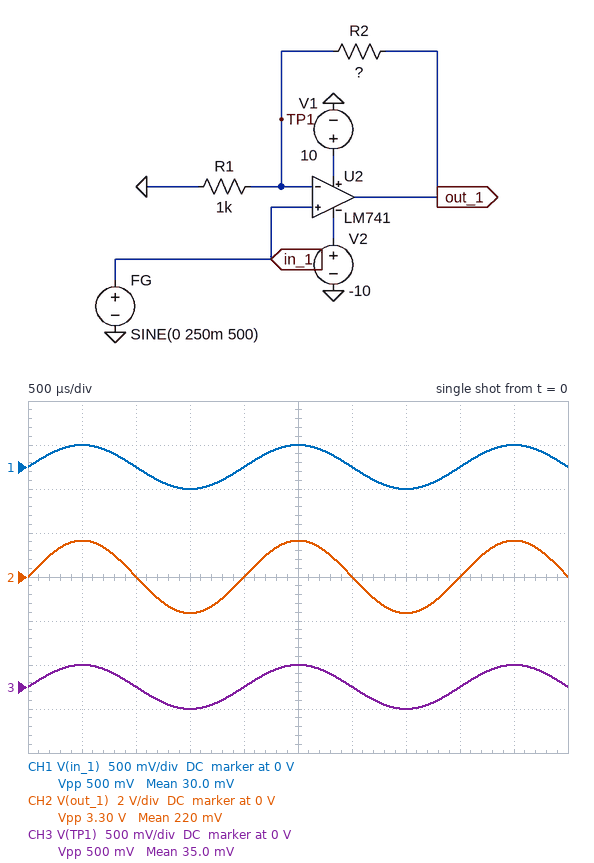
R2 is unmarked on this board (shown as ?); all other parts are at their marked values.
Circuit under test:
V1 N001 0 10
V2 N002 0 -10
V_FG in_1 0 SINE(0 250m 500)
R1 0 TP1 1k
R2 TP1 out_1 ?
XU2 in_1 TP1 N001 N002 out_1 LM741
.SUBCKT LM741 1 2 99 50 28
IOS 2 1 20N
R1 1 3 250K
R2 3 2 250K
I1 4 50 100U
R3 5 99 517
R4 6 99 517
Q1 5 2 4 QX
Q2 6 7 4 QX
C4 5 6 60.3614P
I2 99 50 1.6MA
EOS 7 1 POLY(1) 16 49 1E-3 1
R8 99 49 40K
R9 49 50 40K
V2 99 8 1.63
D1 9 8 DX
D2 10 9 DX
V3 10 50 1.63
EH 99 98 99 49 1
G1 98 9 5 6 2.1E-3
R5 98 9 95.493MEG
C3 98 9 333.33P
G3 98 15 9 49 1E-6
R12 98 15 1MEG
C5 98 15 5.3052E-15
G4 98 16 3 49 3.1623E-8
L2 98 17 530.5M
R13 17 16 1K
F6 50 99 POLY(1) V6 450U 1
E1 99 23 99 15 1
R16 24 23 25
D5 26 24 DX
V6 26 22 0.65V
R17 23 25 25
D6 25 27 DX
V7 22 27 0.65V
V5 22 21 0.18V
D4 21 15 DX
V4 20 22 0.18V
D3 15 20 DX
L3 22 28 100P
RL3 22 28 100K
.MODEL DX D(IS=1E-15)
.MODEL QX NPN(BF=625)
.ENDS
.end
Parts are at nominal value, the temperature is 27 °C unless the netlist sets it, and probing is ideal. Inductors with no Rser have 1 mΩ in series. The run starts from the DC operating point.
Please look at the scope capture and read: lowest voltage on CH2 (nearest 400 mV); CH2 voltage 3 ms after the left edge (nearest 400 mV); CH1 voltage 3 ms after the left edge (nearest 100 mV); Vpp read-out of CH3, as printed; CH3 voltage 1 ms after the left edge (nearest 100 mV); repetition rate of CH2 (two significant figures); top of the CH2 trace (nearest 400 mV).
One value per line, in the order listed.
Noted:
-1.6 V
0 V
0 V
500 mV
0 V
500 Hz
1.6 V
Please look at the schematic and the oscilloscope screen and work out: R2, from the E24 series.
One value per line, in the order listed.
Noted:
5.6 kΩ
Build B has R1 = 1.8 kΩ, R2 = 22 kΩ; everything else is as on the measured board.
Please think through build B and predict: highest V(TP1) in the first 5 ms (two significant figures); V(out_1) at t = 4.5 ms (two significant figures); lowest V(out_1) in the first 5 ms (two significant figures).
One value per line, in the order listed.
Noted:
250 mV
3.3 V
-3.3 V
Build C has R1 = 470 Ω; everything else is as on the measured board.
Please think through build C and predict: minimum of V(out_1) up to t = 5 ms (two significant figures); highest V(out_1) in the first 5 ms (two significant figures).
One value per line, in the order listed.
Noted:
-3.2 V
3.2 V
